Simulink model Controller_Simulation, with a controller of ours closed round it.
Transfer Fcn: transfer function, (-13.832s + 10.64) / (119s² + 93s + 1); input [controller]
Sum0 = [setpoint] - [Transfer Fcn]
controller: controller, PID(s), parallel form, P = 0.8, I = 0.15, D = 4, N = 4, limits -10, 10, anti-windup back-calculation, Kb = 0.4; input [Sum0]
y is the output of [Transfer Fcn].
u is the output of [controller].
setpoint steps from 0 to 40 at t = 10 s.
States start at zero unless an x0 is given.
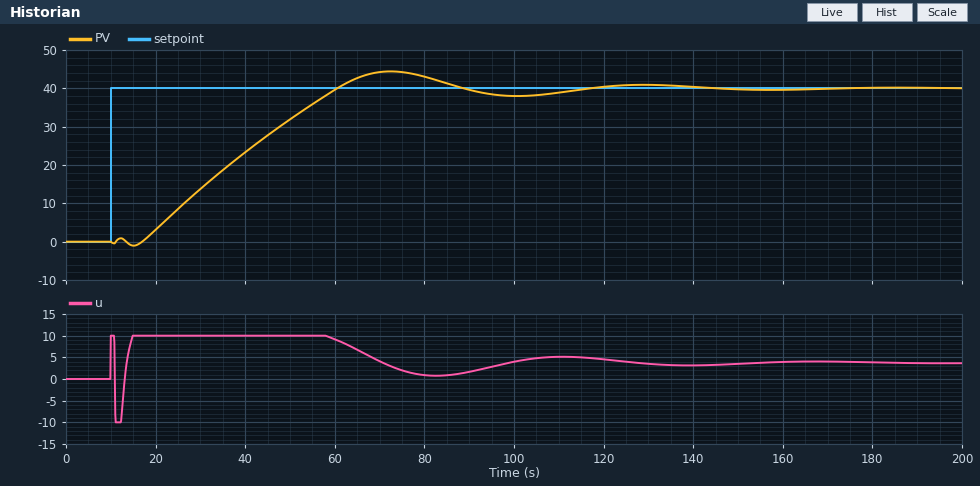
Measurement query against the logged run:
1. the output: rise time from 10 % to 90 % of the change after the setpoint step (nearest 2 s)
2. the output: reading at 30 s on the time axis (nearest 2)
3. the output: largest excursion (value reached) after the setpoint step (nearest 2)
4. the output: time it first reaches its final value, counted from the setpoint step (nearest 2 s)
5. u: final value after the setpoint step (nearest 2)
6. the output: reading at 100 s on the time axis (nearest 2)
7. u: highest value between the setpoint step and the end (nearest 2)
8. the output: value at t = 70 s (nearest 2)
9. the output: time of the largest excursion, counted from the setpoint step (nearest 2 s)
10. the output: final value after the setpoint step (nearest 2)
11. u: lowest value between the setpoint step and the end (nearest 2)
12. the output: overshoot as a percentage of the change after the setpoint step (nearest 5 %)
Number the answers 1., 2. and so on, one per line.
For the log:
1. 34 s
2. 14
3. 44
4. 50 s
5. 4
6. 38
7. 10
8. 44
9. 62 s
10. 40
11. -10
12. 10 %
